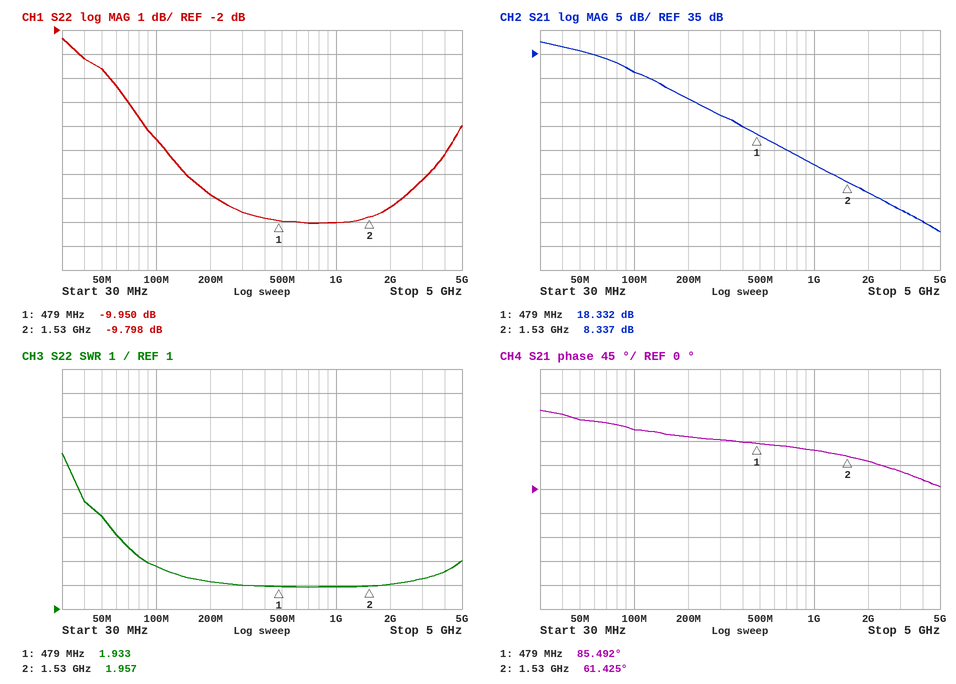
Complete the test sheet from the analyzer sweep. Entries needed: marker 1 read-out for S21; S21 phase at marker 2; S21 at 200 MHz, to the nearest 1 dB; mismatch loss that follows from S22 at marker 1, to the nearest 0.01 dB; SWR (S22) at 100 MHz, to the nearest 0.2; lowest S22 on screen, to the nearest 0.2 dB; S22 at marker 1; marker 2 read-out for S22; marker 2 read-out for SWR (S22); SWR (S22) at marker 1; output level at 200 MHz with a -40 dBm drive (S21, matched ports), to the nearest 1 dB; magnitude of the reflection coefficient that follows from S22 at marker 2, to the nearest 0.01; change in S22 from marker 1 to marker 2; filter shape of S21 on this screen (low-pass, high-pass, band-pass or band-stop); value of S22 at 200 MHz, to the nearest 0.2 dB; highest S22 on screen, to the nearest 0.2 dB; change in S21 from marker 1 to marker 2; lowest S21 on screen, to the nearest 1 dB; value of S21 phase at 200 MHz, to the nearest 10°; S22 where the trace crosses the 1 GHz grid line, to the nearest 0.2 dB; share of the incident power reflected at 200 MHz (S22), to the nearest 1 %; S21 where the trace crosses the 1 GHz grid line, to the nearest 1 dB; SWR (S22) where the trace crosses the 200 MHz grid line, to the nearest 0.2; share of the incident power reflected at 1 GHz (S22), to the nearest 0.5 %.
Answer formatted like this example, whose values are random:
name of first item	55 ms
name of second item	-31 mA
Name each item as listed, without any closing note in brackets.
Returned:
marker 1 read-out for S21	18.332 dB
S21 phase at marker 2	61.425°
S21 at 200 MHz, to the nearest 1 dB	26 dB
mismatch loss that follows from S22 at marker 1, to the nearest 0.01 dB	0.46 dB
SWR (S22) at 100 MHz, to the nearest 0.2	2.8
lowest S22 on screen, to the nearest 0.2 dB	-10.0 dB
S22 at marker 1	-9.950 dB
marker 2 read-out for S22	-9.798 dB
marker 2 read-out for SWR	1.957
SWR (S22) at marker 1	1.933
output level at 200 MHz with a -40 dBm drive (S21, matched ports), to the nearest 1 dB	-14 dBm
magnitude of the reflection coefficient that follows from S22 at marker 2, to the nearest 0.01	0.32
change in S22 from marker 1 to marker 2	0.152 dB
filter shape of S21 on this screen	low-pass
value of S22 at 200 MHz, to the nearest 0.2 dB	-8.8 dB
highest S22 on screen, to the nearest 0.2 dB	-2.4 dB
change in S21 from marker 1 to marker 2	-9.995 dB
lowest S21 on screen, to the nearest 1 dB	-2 dB
value of S21 phase at 200 MHz, to the nearest 10°	100°
S22 where the trace crosses the 1 GHz grid line, to the nearest 0.2 dB	-10.0 dB
share of the incident power reflected at 200 MHz (S22), to the nearest 1 %	13 %
S21 where the trace crosses the 1 GHz grid line, to the nearest 1 dB	12 dB
SWR (S22) where the trace crosses the 200 MHz grid line, to the nearest 0.2	2.2
share of the incident power reflected at 1 GHz (S22), to the nearest 0.5 %	10.0 %
